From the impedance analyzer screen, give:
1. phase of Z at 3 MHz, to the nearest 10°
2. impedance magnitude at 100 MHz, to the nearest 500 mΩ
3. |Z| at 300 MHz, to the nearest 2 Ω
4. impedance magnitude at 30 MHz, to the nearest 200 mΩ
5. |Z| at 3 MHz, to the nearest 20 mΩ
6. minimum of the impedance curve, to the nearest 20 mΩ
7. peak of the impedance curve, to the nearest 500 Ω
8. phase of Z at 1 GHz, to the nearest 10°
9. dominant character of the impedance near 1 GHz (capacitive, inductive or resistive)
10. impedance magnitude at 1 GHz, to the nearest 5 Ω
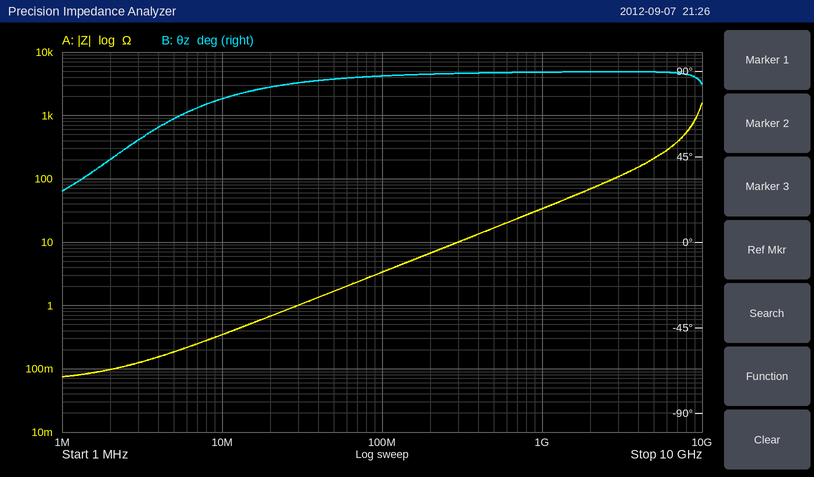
50°
3.5 Ω
10 Ω
1.0 Ω
120 mΩ
80 mΩ
1.5 kΩ
90°
inductive
35 Ω
